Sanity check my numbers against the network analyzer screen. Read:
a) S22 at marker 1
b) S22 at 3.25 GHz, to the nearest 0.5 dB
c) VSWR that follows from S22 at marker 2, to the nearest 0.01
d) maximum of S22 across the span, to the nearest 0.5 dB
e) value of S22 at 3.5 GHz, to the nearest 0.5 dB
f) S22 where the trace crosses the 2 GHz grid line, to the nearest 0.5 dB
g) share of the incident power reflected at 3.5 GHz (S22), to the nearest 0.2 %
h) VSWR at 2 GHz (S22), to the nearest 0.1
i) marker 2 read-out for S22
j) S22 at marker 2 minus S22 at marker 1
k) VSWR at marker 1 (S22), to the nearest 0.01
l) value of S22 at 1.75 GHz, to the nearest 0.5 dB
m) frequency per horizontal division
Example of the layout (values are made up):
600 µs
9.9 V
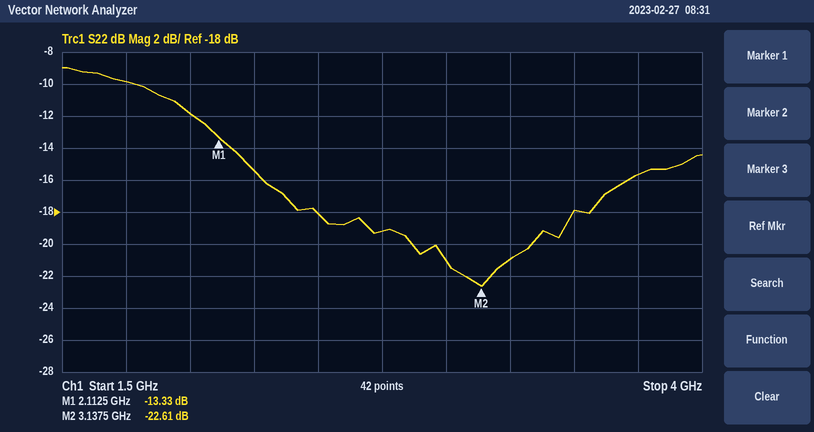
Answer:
-13.33 dB
-21.0 dB
1.16
-9.0 dB
-18.0 dB
-12.0 dB
1.6 %
1.7
-22.61 dB
-9.28 dB
1.55
-10.0 dB
250 MHz
